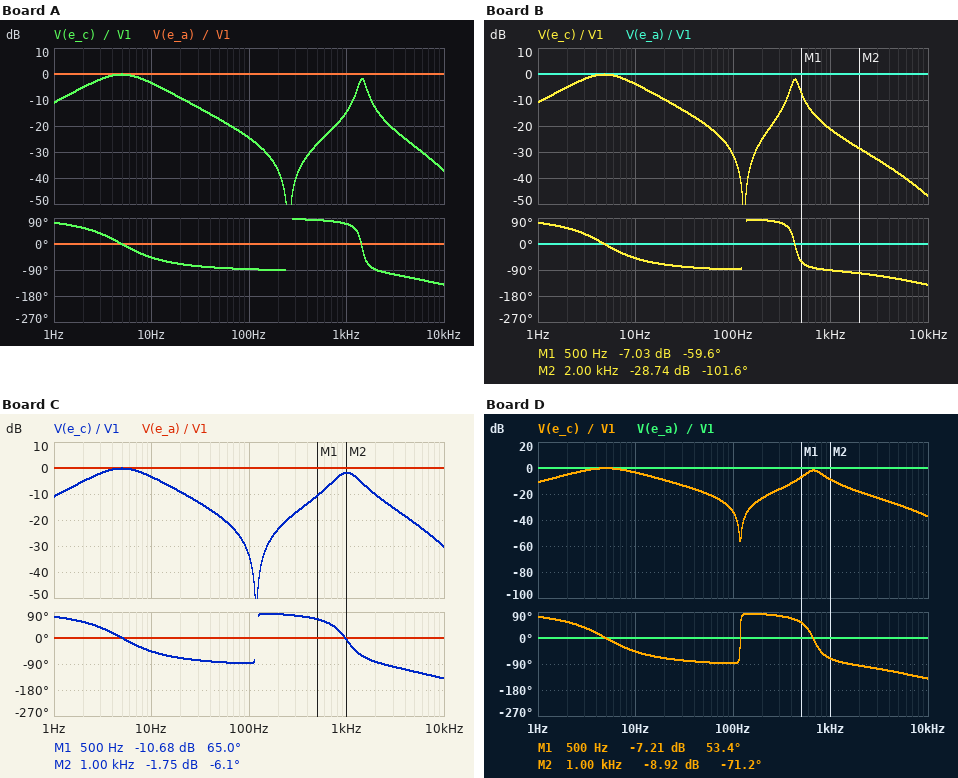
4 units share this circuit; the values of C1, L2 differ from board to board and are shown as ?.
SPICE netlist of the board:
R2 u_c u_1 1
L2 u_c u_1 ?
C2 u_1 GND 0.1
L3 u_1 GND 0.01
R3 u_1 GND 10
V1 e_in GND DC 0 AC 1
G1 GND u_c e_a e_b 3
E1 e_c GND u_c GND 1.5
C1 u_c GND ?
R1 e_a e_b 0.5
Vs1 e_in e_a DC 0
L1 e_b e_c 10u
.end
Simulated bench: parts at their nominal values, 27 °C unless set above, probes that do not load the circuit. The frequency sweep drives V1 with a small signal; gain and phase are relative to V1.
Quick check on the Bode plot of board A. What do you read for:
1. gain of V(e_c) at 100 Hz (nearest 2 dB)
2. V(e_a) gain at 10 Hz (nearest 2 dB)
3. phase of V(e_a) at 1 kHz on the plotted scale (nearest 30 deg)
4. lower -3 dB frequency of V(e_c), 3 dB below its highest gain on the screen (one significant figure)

-24 dB
0 dB
0 deg
3 Hz
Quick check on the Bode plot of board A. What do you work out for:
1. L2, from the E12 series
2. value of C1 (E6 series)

3.9 µH
3.3 mF
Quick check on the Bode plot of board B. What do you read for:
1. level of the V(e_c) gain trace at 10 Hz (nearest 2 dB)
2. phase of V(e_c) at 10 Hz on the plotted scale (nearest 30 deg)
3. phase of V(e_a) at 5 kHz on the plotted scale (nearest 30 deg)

-4 dB
-60 deg
0 deg
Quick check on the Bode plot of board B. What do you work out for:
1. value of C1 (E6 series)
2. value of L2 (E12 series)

10 mF
15 µH
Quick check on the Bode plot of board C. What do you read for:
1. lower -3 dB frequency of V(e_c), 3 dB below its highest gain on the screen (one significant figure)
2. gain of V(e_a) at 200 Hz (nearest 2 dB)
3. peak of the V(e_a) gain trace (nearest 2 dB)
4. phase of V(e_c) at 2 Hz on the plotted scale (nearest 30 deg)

3 Hz
0 dB
0 dB
60 deg
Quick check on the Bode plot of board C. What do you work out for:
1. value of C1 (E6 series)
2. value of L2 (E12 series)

1.5 mF
18 µH
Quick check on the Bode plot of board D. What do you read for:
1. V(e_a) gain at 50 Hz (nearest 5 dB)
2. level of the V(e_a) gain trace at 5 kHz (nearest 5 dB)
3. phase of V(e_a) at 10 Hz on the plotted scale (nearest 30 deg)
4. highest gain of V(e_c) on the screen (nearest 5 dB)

0 dB
0 dB
0 deg
0 dB
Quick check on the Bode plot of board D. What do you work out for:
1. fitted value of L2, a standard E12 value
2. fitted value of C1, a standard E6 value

18 µH
3.3 mF
